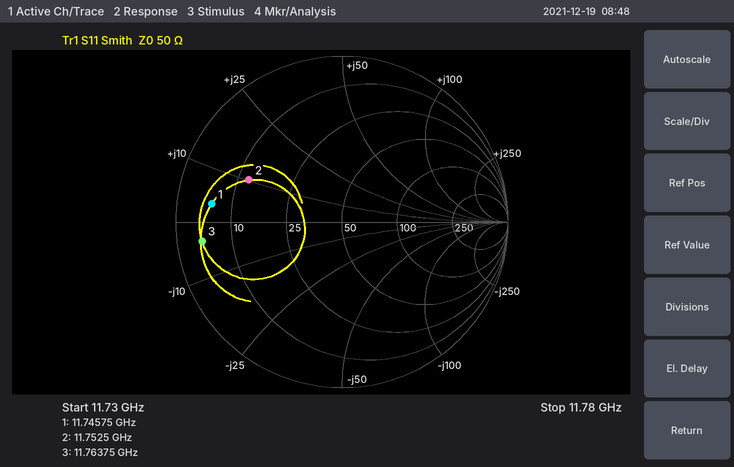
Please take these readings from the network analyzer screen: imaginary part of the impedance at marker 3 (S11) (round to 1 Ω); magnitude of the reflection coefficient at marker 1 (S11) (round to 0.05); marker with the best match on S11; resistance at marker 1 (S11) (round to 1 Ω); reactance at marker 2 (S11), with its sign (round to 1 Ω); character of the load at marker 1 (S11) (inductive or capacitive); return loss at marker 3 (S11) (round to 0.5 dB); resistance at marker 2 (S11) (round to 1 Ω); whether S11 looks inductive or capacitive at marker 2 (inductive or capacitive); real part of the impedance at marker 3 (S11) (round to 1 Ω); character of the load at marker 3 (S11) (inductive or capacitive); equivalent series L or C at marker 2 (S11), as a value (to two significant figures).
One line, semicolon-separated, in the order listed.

-3 Ω; 0.80; marker 2; 6 Ω; +10 Ω; inductive; 1.5 dB; 12 Ω; inductive; 4 Ω; capacitive; 140 pH
